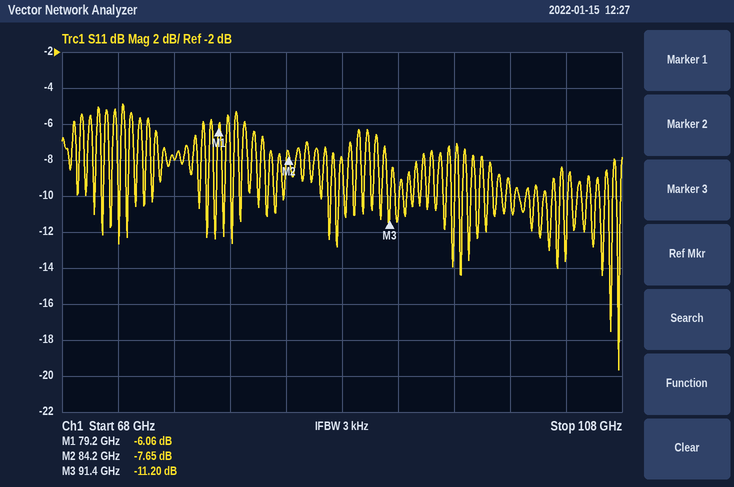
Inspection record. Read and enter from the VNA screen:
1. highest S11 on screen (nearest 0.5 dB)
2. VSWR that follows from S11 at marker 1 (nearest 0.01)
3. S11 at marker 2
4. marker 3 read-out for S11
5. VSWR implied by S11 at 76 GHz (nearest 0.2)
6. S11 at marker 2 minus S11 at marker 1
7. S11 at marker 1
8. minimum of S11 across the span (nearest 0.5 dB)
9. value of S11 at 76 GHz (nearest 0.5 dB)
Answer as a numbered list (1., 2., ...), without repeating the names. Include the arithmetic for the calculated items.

1. -5.0 dB
2. (1 + 0.4977)/(1 − 0.4977) ≈ 2.98
3. -7.65 dB
4. -11.20 dB
5. |Γ| = 10^(-8/20) = 0.3981; VSWR = (1 + 0.3981)/(1 − 0.3981) ≈ 2.32, so 2.4 to the nearest 0.2
6. -7.65 − (-6.06) = -1.59 dB
7. -6.06 dB
8. -19.5 dB
9. -8.0 dB
